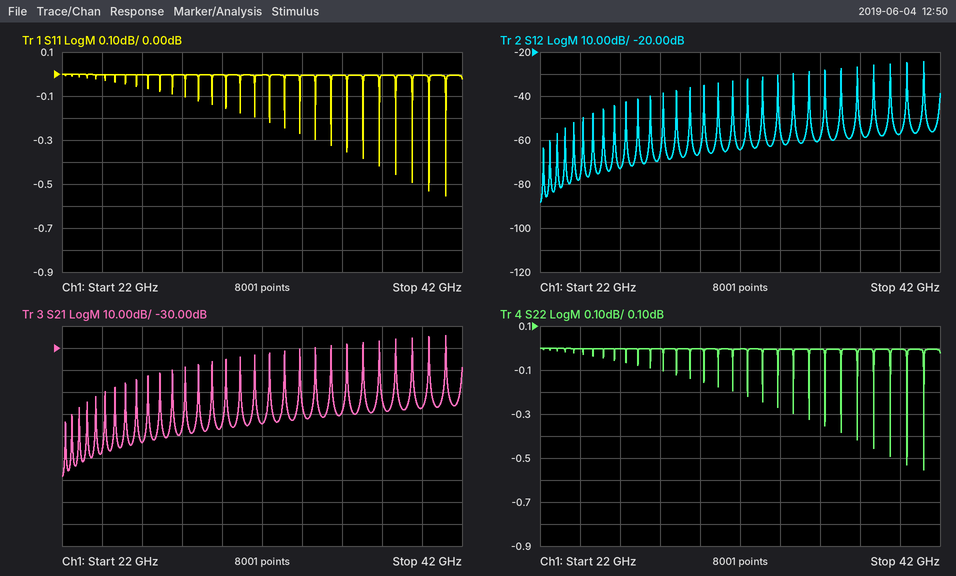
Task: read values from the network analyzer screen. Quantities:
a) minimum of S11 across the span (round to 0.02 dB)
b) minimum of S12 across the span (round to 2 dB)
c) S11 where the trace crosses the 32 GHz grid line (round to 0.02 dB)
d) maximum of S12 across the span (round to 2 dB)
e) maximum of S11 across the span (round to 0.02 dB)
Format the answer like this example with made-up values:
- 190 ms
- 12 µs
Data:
- -0.56 dB
- -88 dB
- 0.00 dB
- -24 dB
- 0.00 dB
